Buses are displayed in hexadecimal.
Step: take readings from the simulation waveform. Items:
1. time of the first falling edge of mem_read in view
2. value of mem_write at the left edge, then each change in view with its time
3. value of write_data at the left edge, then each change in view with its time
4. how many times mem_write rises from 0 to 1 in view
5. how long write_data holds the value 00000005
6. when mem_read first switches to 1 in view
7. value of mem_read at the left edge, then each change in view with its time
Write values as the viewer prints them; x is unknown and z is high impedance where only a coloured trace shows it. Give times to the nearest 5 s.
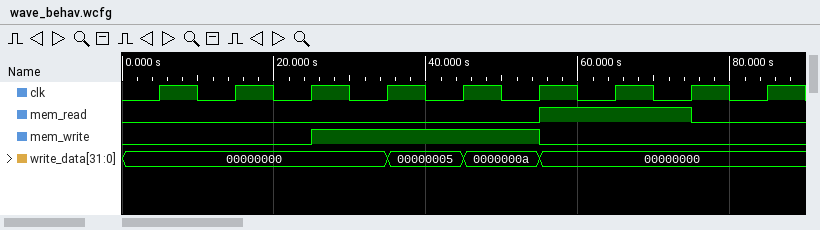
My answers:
75 s
0, 1 at 25 s, 0 at 55 s
00000000, 00000005 at 35 s, 0000000a at 45 s, 00000000 at 55 s
1
10 s
55 s
0, 1 at 55 s, 0 at 75 s
